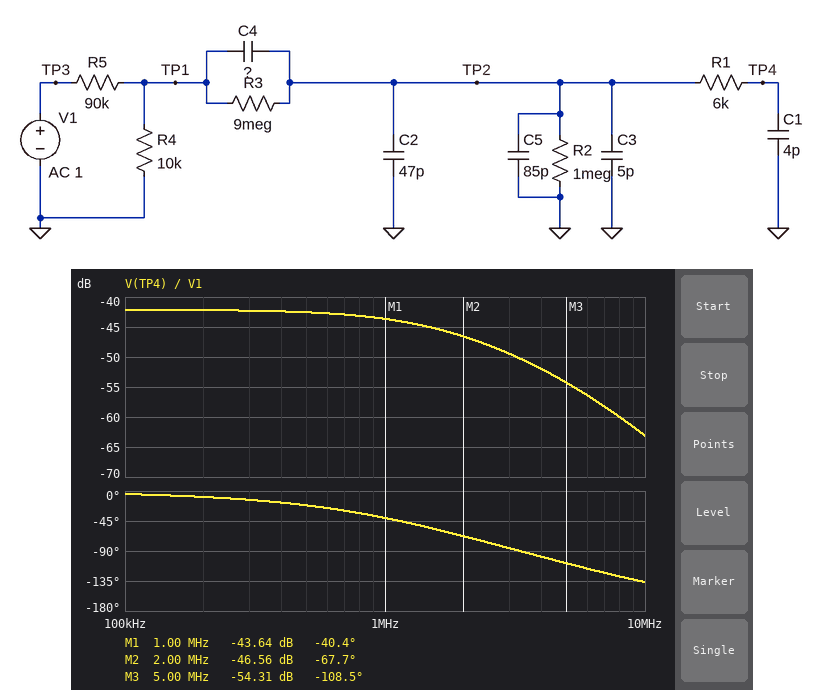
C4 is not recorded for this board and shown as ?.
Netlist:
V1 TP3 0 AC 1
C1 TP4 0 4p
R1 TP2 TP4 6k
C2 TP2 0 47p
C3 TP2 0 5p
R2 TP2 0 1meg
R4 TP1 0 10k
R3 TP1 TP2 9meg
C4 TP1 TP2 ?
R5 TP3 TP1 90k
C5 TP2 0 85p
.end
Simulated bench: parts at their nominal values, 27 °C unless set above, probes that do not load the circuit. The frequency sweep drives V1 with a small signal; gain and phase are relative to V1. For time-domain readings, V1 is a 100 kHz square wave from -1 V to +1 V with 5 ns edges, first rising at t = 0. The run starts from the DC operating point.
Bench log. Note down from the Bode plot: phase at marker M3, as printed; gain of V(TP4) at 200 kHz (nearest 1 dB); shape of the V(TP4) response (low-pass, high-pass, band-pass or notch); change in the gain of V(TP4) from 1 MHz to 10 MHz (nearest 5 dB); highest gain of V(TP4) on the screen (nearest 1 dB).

-108.5 deg
-42 dB
low-pass
-20 dB
-42 dB
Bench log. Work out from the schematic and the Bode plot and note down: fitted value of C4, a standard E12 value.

12 pF
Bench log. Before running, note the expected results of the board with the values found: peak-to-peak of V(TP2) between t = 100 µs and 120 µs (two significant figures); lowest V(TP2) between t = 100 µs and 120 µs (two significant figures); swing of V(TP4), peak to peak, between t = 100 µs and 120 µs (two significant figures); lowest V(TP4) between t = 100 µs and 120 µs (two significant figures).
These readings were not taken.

16 mV
-8.9 mV
16 mV
-8.9 mV
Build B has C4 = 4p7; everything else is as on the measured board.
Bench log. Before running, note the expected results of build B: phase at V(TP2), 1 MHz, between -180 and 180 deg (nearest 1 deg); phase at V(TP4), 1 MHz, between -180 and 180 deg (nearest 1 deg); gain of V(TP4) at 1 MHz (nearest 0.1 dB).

-14 deg
-23 deg
-50.2 dB
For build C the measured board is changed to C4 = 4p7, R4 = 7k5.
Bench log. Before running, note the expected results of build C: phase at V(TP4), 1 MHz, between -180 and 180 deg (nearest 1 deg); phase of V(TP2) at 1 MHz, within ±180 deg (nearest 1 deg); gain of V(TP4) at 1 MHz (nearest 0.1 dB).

-20 deg
-11 deg
-52.4 dB
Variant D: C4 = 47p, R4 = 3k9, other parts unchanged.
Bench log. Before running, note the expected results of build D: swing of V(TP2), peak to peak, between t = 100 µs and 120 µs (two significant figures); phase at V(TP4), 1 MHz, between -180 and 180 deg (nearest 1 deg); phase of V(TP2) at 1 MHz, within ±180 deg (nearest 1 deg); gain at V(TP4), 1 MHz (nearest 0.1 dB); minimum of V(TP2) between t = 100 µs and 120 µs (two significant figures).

21 mV
-48 deg
-39 deg
-42.0 dB
-7.3 mV
